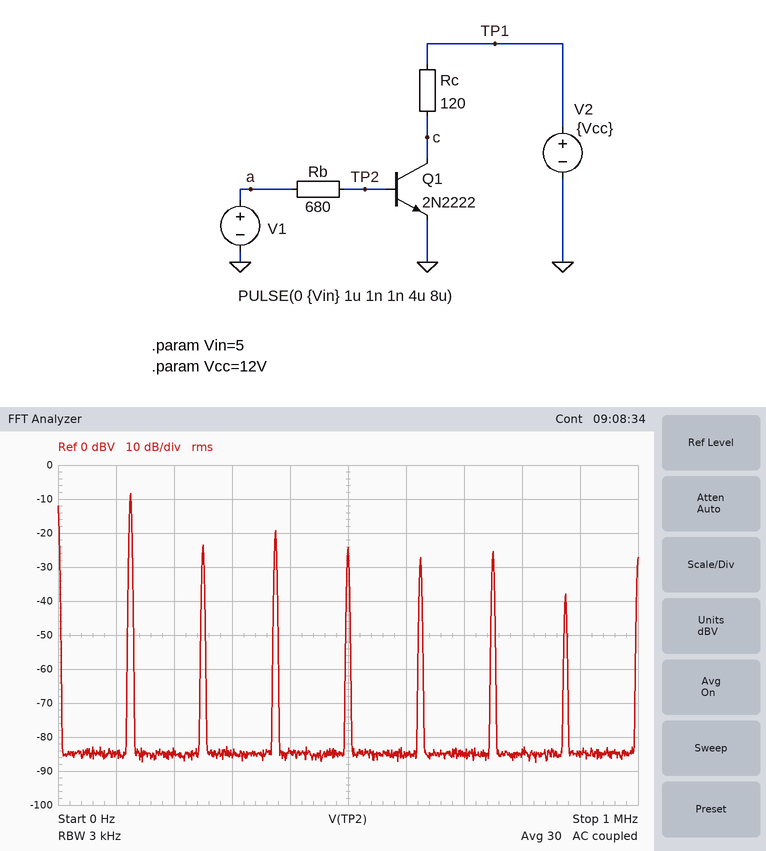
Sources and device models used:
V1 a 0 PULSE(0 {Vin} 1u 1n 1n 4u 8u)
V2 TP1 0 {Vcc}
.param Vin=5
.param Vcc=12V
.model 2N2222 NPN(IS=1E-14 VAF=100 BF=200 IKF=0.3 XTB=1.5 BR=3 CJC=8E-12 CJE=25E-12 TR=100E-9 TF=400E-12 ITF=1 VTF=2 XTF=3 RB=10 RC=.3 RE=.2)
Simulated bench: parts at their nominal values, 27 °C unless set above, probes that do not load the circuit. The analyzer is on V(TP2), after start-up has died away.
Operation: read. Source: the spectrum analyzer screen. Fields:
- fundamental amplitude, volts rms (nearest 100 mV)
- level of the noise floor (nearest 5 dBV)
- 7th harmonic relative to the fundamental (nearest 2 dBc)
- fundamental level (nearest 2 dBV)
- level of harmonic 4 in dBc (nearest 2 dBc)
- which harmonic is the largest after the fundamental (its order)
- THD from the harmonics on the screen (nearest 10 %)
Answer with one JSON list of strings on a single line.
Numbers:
["400 mV", "-85 dBV", "-30 dBc", "-8 dBV", "-16 dBc", "3", "40 %"]
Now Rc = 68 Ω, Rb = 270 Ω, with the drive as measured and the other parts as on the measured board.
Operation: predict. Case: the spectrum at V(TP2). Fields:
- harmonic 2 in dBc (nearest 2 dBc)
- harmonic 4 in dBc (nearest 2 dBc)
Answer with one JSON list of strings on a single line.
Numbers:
["-16 dBc", "-18 dBc"]
